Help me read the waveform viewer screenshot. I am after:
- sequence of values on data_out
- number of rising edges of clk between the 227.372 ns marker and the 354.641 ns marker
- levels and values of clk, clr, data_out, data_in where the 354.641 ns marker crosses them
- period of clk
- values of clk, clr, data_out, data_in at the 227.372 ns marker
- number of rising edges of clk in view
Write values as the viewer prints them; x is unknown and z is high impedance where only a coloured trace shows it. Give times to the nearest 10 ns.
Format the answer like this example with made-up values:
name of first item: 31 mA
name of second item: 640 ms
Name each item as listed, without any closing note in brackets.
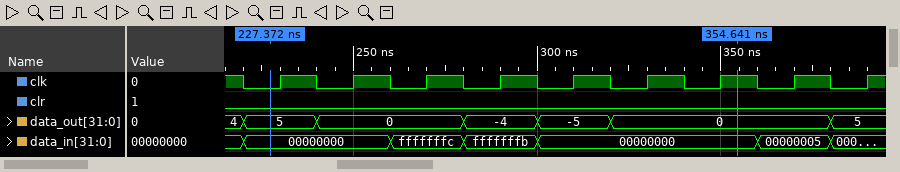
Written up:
sequence of values on data_out: 4, 5, 0, -4, -5, 0, 5
number of rising edges of clk between the 227.372 ns marker and the 354.641 ns marker: 7
levels and values of clk, clr, data_out, data_in where the 354.641 ns marker crosses them: clk=1, clr=0, data_out=0, data_in=00000000
period of clk: 20 ns
values of clk, clr, data_out, data_in at the 227.372 ns marker: clk=0, clr=0, data_out=5, data_in=00000000
number of rising edges of clk in view: 9
